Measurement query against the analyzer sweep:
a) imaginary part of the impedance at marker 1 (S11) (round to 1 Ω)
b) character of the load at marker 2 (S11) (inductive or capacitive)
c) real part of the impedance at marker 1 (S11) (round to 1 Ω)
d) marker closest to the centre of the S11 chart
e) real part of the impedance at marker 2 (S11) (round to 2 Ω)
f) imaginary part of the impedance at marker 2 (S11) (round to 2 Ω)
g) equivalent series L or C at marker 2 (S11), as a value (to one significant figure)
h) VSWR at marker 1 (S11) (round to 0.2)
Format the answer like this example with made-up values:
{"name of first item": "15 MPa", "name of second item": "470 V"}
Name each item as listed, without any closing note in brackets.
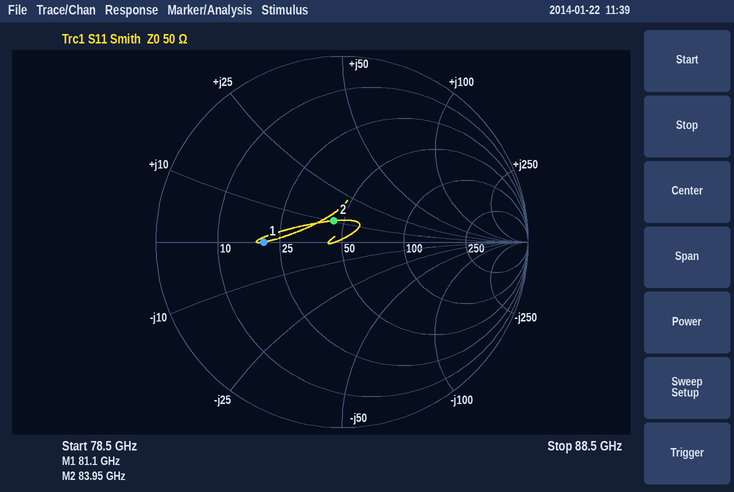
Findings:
{"imaginary part of the impedance at marker 1 (S11)": "0 Ω", "character of the load at marker 2 (S11)": "inductive", "real part of the impedance at marker 1 (S11)": "20 Ω", "marker closest to the centre of the S11 chart": "marker 2", "real part of the impedance at marker 2 (S11)": "44 Ω", "imaginary part of the impedance at marker 2 (S11)": "+10 Ω", "equivalent series L or C at marker 2 (S11), as a value": "20 pH", "VSWR at marker 1 (S11)": "2.4"}
